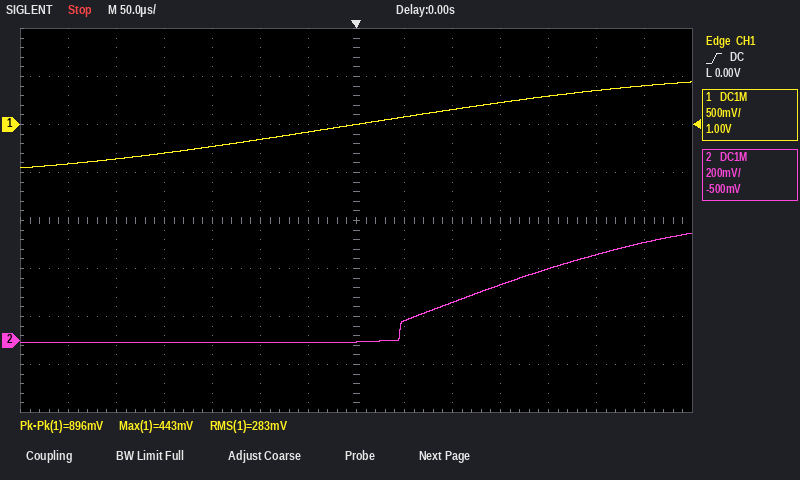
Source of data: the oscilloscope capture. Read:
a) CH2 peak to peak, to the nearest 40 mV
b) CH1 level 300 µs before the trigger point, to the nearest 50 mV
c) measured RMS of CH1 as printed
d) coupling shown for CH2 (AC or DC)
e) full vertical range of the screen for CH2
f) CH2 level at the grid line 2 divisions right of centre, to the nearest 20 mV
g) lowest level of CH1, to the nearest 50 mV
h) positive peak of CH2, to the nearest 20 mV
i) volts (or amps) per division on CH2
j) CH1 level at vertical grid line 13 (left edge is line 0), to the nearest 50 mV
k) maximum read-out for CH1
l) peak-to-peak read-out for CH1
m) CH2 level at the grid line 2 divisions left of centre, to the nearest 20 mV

440 mV
-400 mV
283 mV
DC
1.6 V
160 mV
-450 mV
440 mV
200 mV
400 mV
443 mV
896 mV
0 mV
